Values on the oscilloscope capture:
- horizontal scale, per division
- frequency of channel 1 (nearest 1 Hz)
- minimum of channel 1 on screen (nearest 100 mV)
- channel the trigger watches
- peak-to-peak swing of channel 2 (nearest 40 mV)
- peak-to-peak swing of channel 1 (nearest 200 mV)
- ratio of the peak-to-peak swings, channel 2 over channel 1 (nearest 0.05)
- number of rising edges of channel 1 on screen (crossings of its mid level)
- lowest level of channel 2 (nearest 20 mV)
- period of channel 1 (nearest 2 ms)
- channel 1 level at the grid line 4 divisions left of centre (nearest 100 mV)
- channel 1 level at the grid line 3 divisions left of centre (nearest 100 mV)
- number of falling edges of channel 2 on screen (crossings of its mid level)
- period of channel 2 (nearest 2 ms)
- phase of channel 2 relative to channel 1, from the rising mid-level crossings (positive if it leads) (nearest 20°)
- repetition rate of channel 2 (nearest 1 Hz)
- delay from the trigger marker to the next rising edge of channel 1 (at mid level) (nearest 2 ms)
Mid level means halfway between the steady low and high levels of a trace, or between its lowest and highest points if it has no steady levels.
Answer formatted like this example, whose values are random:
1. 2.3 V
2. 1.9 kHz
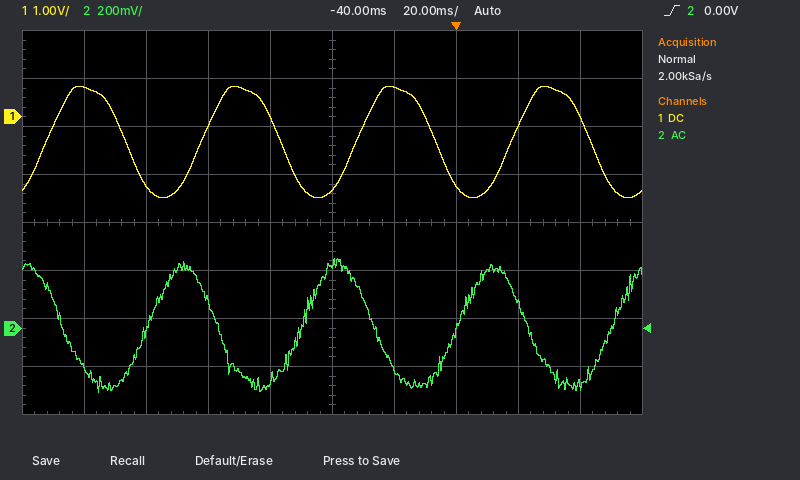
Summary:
1. 20 ms
2. 20 Hz
3. -1.7 V
4. channel 2
5. 560 mV
6. 2.4 V
7. 0.25
8. 4
9. -260 mV
10. 50 ms
11. 600 mV
12. -1.4 V
13. 4
14. 50 ms
15. +120°
16. 20 Hz
17. 18 ms
